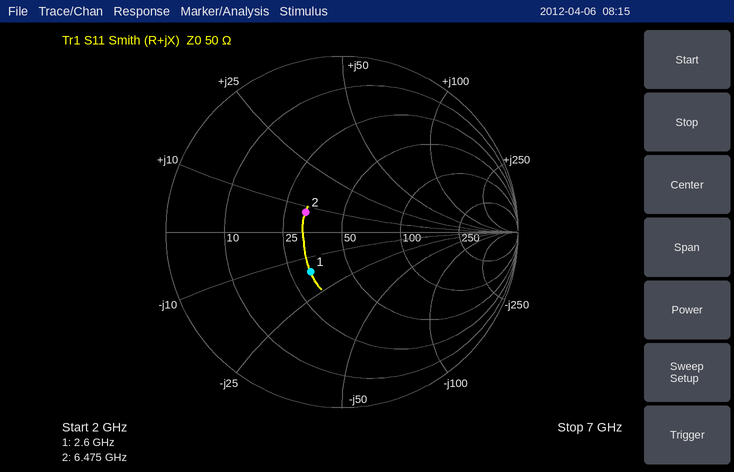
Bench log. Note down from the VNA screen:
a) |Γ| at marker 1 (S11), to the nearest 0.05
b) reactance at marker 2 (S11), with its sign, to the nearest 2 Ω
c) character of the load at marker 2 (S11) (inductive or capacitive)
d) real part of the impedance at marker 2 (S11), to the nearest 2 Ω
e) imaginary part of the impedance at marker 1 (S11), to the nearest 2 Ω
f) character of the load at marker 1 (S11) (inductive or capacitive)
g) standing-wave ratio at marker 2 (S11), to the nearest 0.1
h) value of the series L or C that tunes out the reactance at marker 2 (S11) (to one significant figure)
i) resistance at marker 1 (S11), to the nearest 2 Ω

0.30
+8 Ω
inductive
32 Ω
-16 Ω
capacitive
1.6
3 pF
32 Ω
